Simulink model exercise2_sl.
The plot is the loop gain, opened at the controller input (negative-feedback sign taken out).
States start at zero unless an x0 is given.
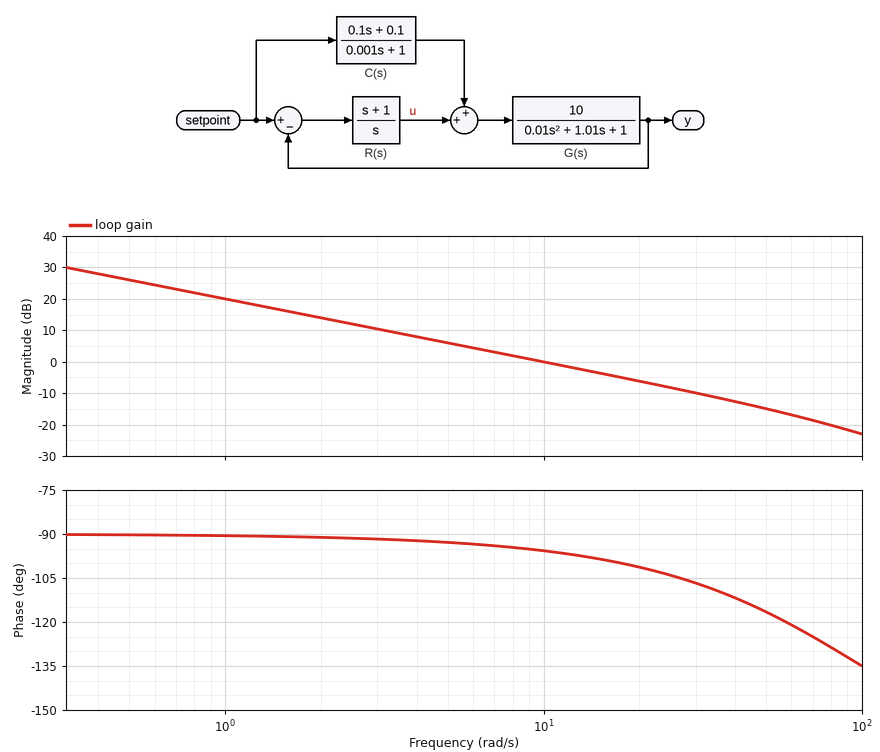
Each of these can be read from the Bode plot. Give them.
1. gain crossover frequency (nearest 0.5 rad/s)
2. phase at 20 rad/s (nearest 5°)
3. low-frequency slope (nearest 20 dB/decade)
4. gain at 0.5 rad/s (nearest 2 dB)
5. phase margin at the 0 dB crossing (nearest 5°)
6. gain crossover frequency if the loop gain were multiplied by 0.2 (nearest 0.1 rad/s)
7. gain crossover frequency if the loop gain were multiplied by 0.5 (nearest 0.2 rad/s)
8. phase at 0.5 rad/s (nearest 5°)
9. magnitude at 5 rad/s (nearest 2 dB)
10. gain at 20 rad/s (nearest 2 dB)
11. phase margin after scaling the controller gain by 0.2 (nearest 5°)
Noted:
10.0 rad/s
-100°
-20 dB/decade
26 dB
85°
2.0 rad/s
5.0 rad/s
-90°
6 dB
-6 dB
90°
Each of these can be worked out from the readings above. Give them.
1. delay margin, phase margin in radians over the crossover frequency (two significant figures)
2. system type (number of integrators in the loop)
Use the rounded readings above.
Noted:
0.15 s
1
